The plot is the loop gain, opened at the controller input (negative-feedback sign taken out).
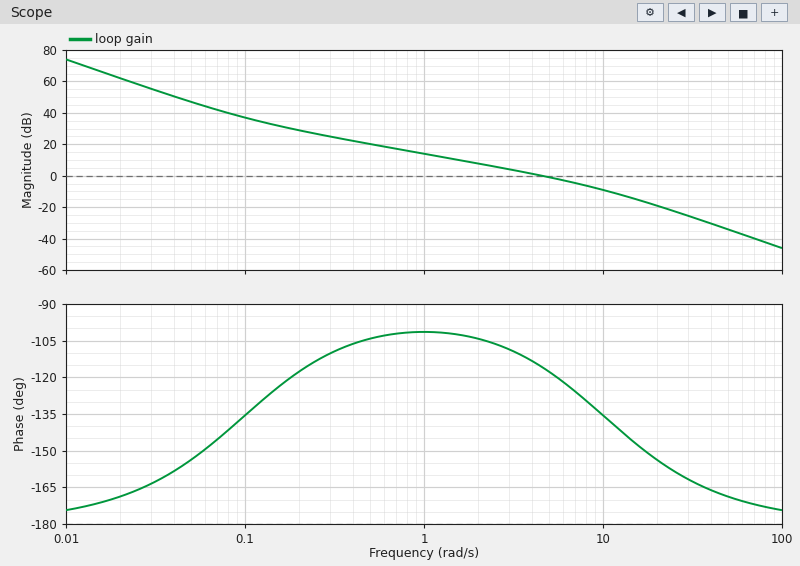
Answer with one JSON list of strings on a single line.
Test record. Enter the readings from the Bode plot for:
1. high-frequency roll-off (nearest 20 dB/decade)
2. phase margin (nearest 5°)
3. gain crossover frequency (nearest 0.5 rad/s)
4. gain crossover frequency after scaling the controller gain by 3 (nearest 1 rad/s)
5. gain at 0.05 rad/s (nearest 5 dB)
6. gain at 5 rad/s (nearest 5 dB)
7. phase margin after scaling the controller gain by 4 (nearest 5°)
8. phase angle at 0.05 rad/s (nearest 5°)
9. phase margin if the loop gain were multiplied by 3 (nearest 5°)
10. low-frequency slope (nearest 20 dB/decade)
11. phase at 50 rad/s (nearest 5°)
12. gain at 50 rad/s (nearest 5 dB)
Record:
["-40 dB/decade", "65°", "4.5 rad/s", "10 rad/s", "45 dB", "0 dB", "40°", "-155°", "45°", "-40 dB/decade", "-170°", "-35 dB"]
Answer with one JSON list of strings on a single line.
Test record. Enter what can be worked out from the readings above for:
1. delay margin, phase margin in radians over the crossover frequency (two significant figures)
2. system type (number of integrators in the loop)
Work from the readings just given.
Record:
["0.25 s", "2"]
